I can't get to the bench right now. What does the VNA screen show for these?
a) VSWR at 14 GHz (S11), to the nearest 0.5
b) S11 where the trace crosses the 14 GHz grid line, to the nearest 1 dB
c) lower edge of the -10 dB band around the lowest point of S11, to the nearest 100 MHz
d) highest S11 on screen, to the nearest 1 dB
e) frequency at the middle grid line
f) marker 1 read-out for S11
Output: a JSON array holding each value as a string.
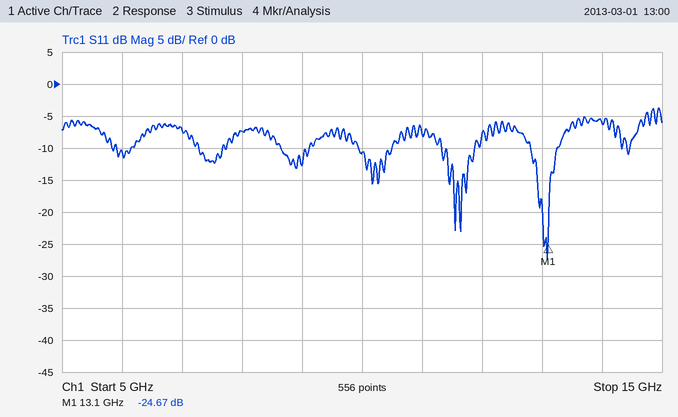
["3.0", "-6 dB", "12.8 GHz", "-4 dB", "10 GHz", "-24.67 dB"]
